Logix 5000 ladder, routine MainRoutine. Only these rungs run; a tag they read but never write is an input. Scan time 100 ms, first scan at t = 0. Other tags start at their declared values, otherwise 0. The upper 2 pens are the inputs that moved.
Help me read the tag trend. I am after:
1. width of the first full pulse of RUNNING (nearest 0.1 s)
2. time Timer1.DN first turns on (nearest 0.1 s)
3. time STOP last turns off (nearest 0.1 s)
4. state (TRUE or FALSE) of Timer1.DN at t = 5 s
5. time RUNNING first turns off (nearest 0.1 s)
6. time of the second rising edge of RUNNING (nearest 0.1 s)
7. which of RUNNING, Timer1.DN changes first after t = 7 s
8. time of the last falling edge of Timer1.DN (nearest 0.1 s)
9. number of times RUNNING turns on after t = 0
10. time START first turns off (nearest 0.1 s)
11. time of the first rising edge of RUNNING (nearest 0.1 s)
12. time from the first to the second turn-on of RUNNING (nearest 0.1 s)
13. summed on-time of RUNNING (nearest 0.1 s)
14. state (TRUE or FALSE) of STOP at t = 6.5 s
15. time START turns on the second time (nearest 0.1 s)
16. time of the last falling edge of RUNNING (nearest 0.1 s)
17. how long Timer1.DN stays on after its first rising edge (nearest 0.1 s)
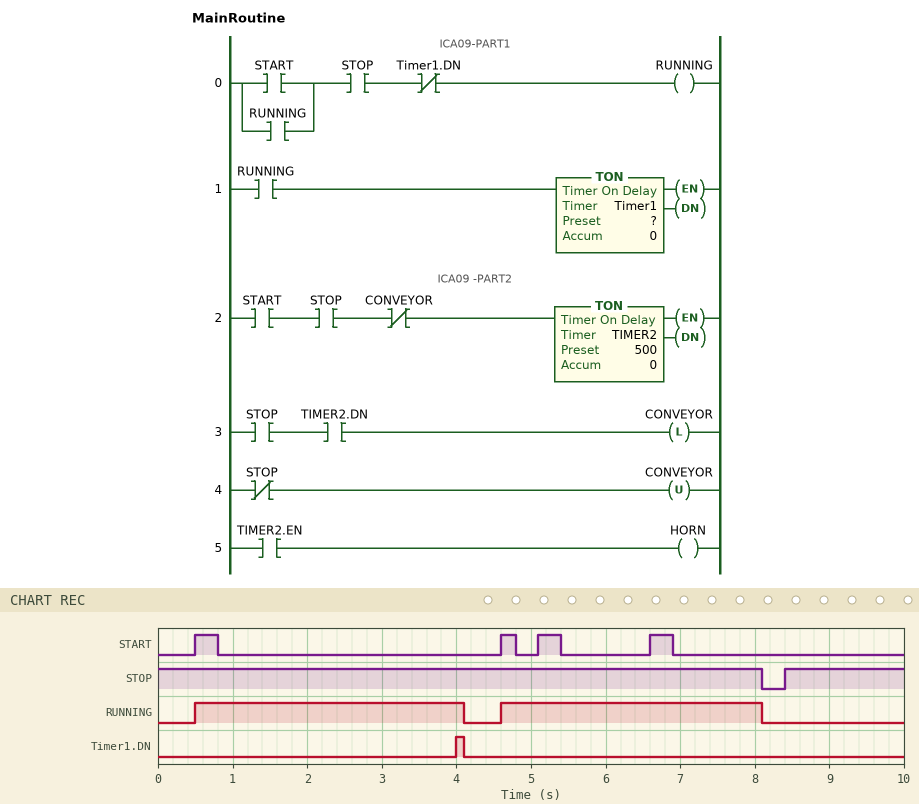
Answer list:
3.6 s
4.0 s
8.1 s
FALSE
4.1 s
4.6 s
RUNNING
4.1 s
2
0.8 s
0.5 s
4.1 s
7.1 s
TRUE
4.6 s
8.1 s
0.1 s
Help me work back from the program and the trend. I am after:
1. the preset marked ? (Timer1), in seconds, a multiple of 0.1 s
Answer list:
3.5 s
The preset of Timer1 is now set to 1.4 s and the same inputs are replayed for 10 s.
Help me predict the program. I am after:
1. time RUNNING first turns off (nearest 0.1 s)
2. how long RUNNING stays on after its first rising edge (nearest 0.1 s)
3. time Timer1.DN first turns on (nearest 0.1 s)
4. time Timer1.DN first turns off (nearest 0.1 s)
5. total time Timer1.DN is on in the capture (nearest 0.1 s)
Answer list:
2.0 s
1.5 s
1.9 s
2.0 s
0.3 s
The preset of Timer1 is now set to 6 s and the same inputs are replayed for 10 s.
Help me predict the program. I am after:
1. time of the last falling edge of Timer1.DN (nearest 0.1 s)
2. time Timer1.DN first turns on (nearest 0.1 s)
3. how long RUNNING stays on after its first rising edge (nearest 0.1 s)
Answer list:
6.6 s
6.5 s
6.1 s
